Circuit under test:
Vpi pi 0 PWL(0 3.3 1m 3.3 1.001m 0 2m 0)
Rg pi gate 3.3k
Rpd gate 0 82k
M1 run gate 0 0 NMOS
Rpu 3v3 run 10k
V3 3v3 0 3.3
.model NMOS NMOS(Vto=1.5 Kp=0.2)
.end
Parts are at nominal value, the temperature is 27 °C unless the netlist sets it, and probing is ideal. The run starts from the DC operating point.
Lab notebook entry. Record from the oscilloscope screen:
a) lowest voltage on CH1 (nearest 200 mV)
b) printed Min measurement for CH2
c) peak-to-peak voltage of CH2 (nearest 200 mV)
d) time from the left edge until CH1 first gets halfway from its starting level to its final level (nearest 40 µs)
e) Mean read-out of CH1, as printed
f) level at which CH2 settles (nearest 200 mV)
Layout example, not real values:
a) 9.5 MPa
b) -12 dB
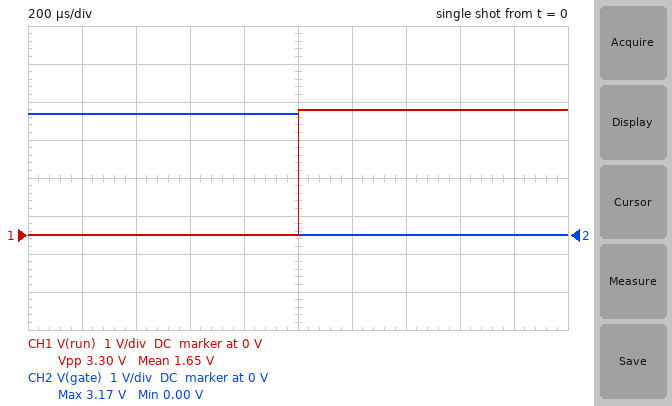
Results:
a) 0 V
b) 0.00 V
c) 3.2 V
d) 1.00 ms
e) 1.65 V
f) 0 V
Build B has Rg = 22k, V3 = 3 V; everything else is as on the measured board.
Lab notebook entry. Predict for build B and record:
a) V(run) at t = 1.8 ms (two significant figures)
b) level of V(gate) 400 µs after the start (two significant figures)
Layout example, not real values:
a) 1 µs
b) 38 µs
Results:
a) 3.0 V
b) 2.6 V
